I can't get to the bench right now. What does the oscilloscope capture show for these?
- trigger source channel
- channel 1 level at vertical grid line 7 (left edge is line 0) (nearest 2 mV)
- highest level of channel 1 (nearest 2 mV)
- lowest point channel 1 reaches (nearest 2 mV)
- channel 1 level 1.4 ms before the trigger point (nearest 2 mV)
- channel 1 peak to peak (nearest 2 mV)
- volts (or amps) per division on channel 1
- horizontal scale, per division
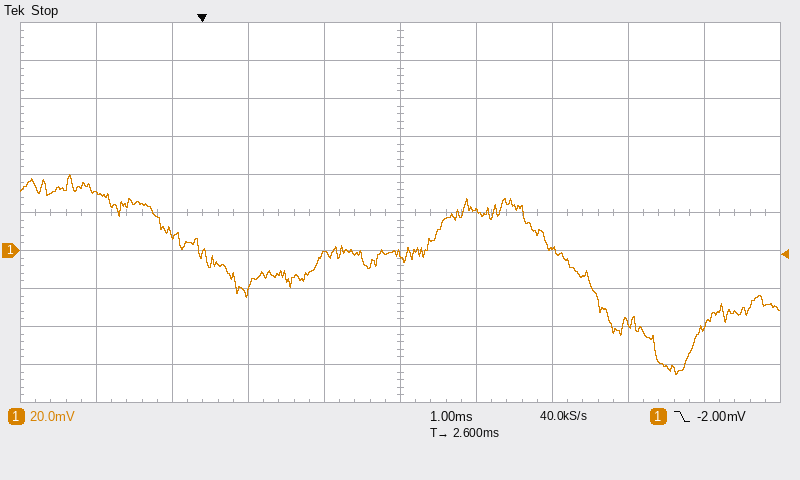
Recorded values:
channel 1
0 mV
40 mV
-66 mV
30 mV
106 mV
20 mV
1 ms
